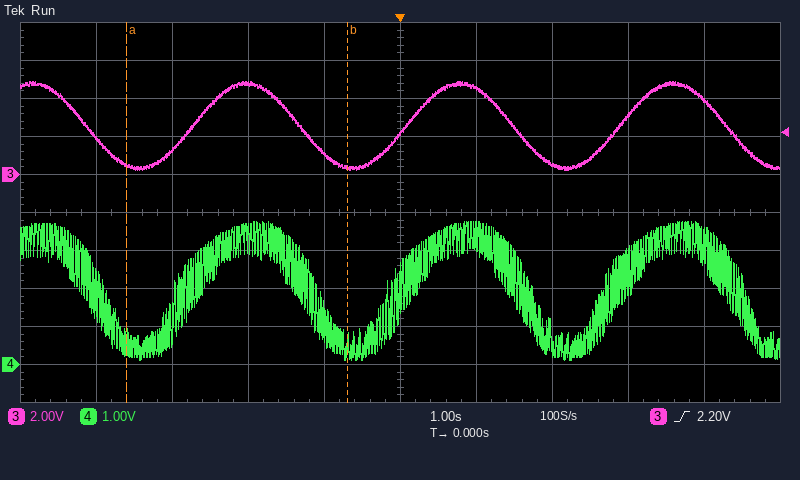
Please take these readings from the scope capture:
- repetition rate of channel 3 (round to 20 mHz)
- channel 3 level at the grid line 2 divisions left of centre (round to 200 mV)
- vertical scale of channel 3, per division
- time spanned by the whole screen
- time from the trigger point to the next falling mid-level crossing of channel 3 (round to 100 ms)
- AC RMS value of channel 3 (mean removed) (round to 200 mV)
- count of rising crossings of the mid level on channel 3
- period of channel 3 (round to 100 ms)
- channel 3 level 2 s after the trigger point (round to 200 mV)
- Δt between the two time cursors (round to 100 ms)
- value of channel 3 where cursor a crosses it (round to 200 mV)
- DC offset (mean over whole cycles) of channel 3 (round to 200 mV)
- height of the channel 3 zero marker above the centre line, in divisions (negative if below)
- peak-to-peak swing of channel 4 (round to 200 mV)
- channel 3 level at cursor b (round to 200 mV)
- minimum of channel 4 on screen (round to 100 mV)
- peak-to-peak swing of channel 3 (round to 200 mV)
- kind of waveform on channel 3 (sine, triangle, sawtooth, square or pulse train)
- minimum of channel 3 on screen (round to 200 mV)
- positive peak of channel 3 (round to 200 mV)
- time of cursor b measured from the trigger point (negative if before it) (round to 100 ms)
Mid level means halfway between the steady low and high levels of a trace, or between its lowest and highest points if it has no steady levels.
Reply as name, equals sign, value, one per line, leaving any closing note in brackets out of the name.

repetition rate of channel 3 = 360 mHz
channel 3 level at the grid line 2 divisions left of centre = 4.8 V
vertical scale of channel 3, per division = 2 V
time spanned by the whole screen = 10 s
time from the trigger point to the next falling mid-level crossing of channel 3 = 1.5 s
AC RMS value of channel 3 (mean removed) = 1.6 V
count of rising crossings of the mid level on channel 3 = 3
period of channel 3 = 2.8 s
channel 3 level 2 s after the trigger point = 600 mV
Δt between the two time cursors = 2.9 s
value of channel 3 where cursor a crosses it = 600 mV
DC offset (mean over whole cycles) of channel 3 = 2.6 V
height of the channel 3 zero marker above the centre line, in divisions = +1.0 div
peak-to-peak swing of channel 4 = 3.6 V
channel 3 level at cursor b = 400 mV
minimum of channel 4 on screen = 100 mV
peak-to-peak swing of channel 3 = 4.6 V
kind of waveform on channel 3 = sine
minimum of channel 3 on screen = 200 mV
positive peak of channel 3 = 4.8 V
time of cursor b measured from the trigger point (negative if before it) = -700 ms
